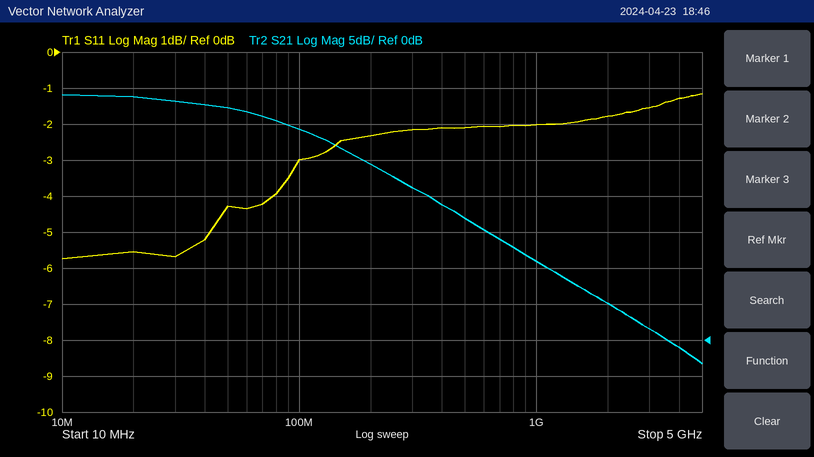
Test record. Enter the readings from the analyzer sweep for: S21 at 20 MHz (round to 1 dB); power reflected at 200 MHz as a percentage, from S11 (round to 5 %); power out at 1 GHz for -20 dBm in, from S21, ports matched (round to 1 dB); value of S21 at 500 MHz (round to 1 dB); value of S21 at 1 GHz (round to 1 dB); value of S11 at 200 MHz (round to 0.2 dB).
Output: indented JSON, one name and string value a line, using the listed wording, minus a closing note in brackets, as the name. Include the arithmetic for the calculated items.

{
  "S21 at 20 MHz": "34 dB",
  "power reflected at 200 MHz as a percentage, from S11": "10^(-2.4/10) ≈ 57.5 %, so 60 % to the nearest 5 %",
  "power out at 1 GHz for -20 dBm in, from S21, ports matched": "-20 dBm + (11 dB) = -9 dBm",
  "value of S21 at 500 MHz": "17 dB",
  "value of S21 at 1 GHz": "11 dB",
  "value of S11 at 200 MHz": "-2.4 dB"
}
